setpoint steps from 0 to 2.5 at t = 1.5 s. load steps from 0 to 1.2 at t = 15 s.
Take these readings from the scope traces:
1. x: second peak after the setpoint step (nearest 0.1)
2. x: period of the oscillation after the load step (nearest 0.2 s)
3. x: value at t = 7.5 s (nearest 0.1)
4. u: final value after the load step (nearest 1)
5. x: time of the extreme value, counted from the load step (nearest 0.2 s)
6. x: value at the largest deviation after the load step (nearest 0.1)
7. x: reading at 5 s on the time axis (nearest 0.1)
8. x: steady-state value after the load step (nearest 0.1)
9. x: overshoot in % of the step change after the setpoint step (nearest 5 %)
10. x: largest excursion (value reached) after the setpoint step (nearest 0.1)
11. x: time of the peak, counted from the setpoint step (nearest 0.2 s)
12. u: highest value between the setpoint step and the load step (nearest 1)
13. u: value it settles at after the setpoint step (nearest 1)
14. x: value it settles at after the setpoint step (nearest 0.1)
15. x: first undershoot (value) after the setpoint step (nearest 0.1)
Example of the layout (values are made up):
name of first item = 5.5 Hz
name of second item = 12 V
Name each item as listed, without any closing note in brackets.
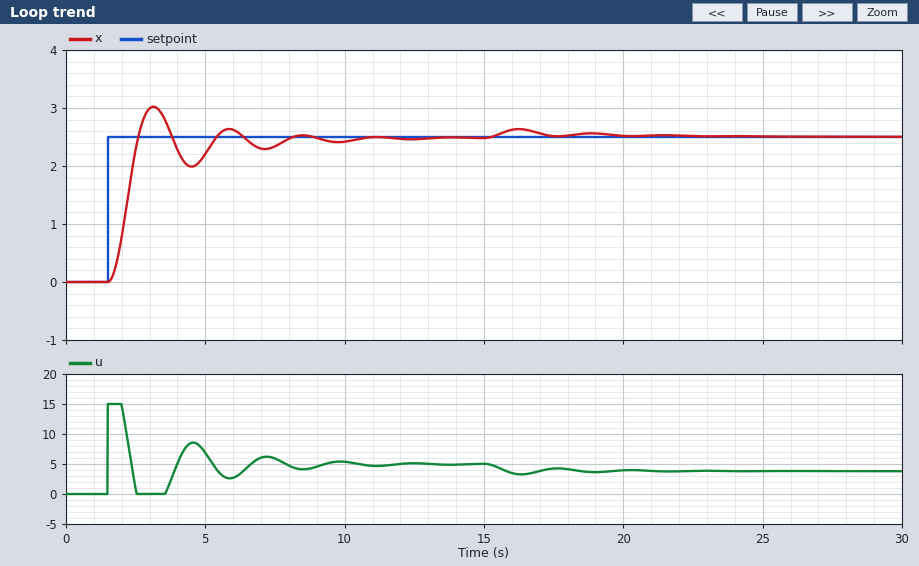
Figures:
x: second peak after the setpoint step = 2.6
x: period of the oscillation after the load step = 2.6 s
x: value at t = 7.5 s = 2.3
u: final value after the load step = 4
x: time of the extreme value, counted from the load step = 1.2 s
x: value at the largest deviation after the load step = 2.6
x: reading at 5 s on the time axis = 2.2
x: steady-state value after the load step = 2.5
x: overshoot in % of the step change after the setpoint step = 20 %
x: largest excursion (value reached) after the setpoint step = 3.0
x: time of the peak, counted from the setpoint step = 1.6 s
u: highest value between the setpoint step and the load step = 15
u: value it settles at after the setpoint step = 5
x: value it settles at after the setpoint step = 2.5
x: first undershoot (value) after the setpoint step = 2.0
